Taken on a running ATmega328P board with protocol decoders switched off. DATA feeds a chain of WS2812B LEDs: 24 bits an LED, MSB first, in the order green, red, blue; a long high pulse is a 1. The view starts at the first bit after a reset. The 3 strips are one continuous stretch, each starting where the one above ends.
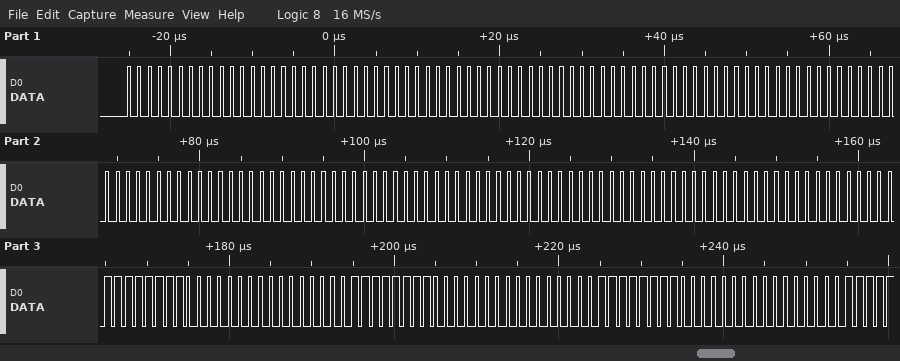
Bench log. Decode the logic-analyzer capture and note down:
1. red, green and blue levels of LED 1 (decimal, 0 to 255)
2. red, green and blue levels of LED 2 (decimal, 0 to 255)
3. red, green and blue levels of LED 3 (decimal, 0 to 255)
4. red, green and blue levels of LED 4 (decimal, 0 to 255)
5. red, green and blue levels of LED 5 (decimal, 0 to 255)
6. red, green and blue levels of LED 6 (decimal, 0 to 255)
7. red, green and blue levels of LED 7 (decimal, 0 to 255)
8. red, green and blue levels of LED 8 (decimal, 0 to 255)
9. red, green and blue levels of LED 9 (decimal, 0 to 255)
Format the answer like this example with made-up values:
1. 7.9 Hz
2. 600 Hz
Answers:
1. 0, 0, 0
2. 0, 0, 0
3. 0, 0, 0
4. 0, 0, 0
5. 0, 0, 0
6. 0, 0, 0
7. 255, 0, 0
8. 255, 0, 0
9. 255, 0, 0
